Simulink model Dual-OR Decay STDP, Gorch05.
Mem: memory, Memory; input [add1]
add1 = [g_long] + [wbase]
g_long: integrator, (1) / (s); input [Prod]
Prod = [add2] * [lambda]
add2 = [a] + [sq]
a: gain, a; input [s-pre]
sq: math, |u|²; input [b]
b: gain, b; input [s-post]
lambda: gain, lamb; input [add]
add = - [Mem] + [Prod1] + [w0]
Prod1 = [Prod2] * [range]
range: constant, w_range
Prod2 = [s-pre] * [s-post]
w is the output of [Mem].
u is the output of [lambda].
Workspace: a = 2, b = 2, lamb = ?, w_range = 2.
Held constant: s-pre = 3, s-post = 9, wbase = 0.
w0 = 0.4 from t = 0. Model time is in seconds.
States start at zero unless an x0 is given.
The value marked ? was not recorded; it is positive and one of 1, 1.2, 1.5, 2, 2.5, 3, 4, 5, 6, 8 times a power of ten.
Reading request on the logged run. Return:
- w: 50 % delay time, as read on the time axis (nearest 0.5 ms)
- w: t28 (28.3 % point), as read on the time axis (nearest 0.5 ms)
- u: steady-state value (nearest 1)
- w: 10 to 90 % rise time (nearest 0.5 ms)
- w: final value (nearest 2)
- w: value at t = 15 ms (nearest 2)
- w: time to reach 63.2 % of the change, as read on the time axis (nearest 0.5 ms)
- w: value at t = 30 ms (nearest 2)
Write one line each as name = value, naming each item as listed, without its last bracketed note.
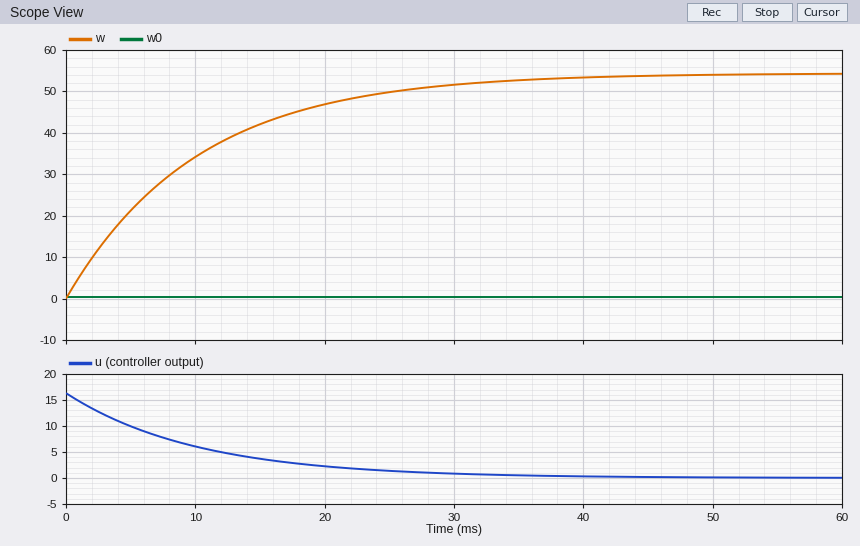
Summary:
w: 50 % delay time, as read on the time axis = 7.0 ms
w: t28 (28.3 % point), as read on the time axis = 3.5 ms
u: steady-state value = 0
w: 10 to 90 % rise time = 22.0 ms
w: final value = 54
w: value at t = 15 ms = 42
w: time to reach 63.2 % of the change, as read on the time axis = 10.0 ms
w: value at t = 30 ms = 52
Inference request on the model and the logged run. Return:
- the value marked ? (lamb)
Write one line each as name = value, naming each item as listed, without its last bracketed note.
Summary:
the value marked ? = 0.3
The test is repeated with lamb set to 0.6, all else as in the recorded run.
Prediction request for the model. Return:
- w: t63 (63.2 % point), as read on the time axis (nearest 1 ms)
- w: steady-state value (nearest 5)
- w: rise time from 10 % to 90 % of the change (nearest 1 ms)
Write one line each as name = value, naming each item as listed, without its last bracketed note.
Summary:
w: t63 (63.2 % point), as read on the time axis = 5 ms
w: steady-state value = 55
w: rise time from 10 % to 90 % of the change = 11 ms
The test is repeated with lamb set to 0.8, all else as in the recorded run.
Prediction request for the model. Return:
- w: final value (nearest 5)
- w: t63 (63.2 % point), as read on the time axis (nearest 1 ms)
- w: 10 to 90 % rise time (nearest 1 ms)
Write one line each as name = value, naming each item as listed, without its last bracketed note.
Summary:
w: final value = 55
w: t63 (63.2 % point), as read on the time axis = 4 ms
w: 10 to 90 % rise time = 8 ms
